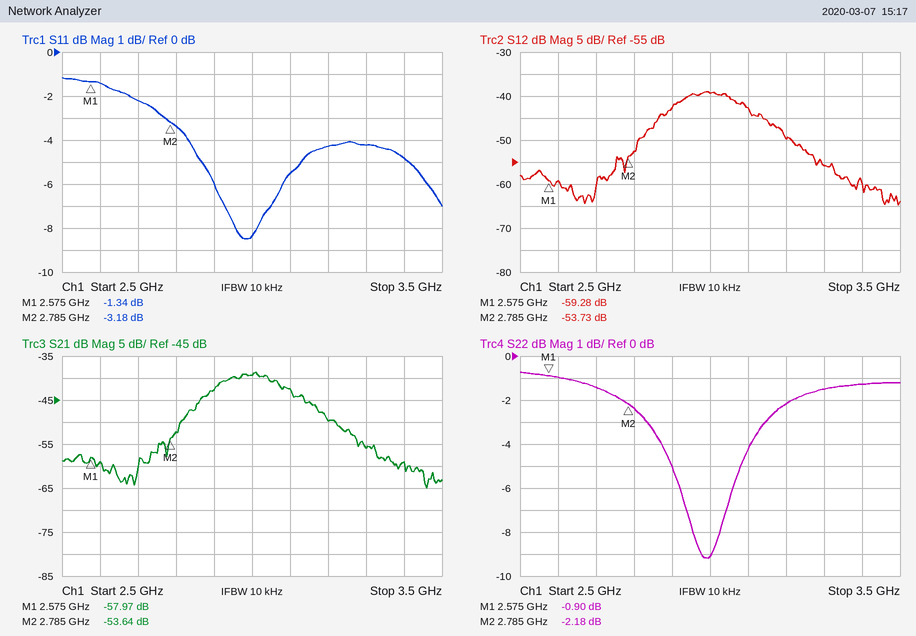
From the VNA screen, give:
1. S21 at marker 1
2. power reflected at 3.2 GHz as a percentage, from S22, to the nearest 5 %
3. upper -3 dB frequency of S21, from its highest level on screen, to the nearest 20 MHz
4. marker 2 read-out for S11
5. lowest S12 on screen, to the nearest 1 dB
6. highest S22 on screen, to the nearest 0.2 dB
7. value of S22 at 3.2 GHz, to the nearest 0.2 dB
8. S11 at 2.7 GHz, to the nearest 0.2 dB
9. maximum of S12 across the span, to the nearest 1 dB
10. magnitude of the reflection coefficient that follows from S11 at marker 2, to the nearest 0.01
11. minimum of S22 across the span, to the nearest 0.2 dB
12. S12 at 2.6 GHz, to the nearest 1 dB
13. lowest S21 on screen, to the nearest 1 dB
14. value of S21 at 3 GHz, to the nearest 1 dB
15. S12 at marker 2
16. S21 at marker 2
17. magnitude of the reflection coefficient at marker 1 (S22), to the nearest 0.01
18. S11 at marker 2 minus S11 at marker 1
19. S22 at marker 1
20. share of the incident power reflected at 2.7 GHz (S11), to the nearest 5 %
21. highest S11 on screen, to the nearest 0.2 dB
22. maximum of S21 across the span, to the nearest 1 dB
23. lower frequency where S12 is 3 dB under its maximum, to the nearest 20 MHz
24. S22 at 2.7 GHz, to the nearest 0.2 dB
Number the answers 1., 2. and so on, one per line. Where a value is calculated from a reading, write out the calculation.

1. -57.97 dB
2. 10^(-2.2/10) ≈ 60 %
3. 3.08 GHz
4. -3.18 dB
5. -65 dB
6. -0.8 dB
7. -2.2 dB
8. -2.2 dB
9. -39 dB
10. 10^(-3.18/20) ≈ 0.69
11. -9.2 dB
12. -59 dB
13. -65 dB
14. -39 dB
15. -53.73 dB
16. -53.64 dB
17. 10^(-0.9/20) ≈ 0.90
18. -3.18 − (-1.34) = -1.84 dB
19. -0.90 dB
20. 10^(-2.2/10) ≈ 60 %
21. -1.2 dB
22. -39 dB
23. 2.90 GHz
24. -1.4 dB
